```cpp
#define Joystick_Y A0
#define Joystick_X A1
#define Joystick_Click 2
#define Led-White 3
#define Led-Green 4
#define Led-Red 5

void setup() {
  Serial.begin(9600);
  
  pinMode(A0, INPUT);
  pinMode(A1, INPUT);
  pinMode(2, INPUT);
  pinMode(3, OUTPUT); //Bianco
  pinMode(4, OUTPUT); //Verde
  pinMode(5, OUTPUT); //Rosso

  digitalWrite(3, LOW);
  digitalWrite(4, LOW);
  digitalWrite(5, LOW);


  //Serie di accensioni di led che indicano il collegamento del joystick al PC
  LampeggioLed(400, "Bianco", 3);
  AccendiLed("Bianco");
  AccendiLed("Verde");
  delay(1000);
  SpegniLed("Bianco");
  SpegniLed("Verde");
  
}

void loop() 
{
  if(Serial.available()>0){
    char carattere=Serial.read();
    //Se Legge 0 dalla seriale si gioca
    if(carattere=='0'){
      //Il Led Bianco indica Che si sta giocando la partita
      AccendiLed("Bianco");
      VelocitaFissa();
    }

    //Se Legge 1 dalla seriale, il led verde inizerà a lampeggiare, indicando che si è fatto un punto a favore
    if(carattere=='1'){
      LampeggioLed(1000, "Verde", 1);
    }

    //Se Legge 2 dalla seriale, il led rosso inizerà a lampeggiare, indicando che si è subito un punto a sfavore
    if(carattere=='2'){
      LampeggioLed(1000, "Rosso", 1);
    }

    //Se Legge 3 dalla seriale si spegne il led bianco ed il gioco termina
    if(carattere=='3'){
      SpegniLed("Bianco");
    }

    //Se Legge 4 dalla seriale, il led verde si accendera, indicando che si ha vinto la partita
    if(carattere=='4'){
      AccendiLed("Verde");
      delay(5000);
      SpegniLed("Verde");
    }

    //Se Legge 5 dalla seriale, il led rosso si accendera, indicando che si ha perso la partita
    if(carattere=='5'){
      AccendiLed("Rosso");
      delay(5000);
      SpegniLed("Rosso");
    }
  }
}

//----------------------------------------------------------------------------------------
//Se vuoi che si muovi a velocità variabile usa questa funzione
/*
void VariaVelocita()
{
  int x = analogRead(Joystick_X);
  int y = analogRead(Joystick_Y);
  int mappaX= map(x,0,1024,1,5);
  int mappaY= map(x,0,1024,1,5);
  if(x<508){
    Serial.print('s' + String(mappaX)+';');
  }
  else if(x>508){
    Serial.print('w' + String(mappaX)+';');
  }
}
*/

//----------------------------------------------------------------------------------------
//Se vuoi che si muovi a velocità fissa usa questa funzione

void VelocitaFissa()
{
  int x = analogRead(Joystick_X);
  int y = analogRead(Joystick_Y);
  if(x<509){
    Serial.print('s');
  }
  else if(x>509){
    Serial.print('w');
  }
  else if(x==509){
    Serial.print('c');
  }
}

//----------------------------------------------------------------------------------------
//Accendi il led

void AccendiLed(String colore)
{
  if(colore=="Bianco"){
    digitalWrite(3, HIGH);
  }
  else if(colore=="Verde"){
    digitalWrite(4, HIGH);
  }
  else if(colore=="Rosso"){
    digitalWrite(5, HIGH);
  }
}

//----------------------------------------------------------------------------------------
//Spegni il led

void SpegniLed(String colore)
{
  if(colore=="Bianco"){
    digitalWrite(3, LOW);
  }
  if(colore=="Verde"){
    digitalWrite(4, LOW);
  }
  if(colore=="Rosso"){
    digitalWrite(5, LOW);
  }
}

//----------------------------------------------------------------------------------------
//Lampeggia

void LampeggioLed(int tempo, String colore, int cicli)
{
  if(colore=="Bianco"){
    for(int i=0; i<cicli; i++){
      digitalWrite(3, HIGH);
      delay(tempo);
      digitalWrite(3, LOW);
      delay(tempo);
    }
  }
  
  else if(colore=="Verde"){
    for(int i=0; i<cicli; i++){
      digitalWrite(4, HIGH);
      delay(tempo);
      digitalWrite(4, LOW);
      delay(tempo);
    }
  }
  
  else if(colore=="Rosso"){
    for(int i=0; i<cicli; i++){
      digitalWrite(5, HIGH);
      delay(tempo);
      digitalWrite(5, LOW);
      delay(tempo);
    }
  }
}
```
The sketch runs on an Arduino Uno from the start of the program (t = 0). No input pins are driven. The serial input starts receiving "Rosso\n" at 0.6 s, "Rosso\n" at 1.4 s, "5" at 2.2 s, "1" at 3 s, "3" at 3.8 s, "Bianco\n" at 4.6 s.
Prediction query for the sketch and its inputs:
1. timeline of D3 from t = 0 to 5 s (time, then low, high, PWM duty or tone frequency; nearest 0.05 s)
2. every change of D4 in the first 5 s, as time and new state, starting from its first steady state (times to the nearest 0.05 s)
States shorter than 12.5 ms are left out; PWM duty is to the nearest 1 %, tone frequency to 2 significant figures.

0 s high; 0.4 s low; 0.8 s high; 1.2 s low; 1.6 s high; 2 s low; 2.4 s high; 3.4 s low
0 s low; 2.4 s high; 3.4 s low
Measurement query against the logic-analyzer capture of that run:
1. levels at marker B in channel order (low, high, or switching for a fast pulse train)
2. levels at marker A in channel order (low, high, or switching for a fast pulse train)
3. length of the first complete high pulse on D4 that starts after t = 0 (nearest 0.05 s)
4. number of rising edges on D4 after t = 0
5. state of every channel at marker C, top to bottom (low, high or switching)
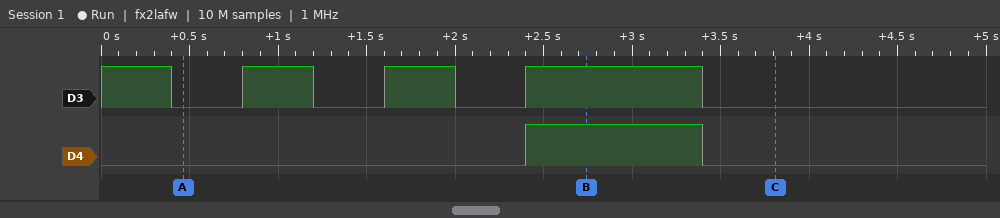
D3 high, D4 high
D3 low, D4 low
1.00 s
1
D3 low, D4 low
